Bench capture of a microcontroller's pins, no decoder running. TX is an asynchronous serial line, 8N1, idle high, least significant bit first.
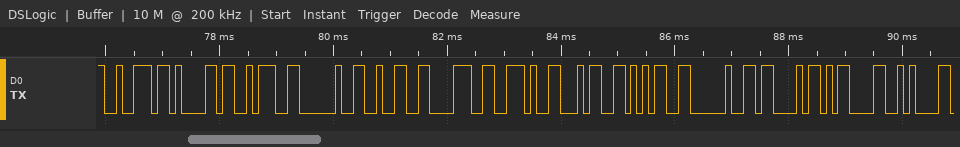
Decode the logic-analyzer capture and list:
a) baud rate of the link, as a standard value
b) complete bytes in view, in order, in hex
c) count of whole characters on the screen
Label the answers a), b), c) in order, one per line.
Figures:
a) 9600 baud
b) 0x72 0x61 0x3A 0x20 0x32 0x38 0x2E 0x34 0x35 0x20 0x43 0x0D 0x0A
c) 13
